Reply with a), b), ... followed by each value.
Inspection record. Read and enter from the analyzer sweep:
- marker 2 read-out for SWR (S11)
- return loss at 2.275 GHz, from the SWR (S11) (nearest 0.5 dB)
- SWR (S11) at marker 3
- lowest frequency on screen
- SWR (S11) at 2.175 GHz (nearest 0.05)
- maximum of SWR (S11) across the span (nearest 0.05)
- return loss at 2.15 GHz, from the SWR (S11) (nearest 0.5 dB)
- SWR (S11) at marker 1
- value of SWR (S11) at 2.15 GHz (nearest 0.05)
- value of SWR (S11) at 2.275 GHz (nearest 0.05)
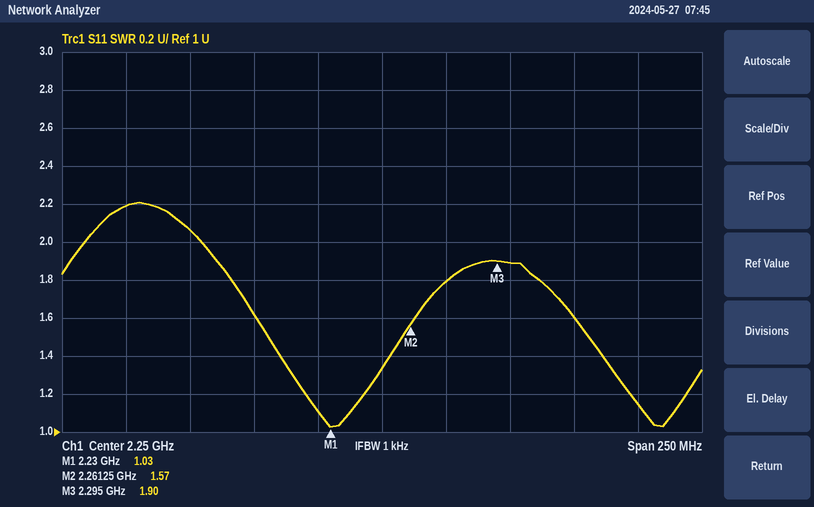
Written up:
a) 1.57
b) 11.0 dB
c) 1.90
d) 2.125 GHz
e) 2.05
f) 2.20
g) 8.5 dB
h) 1.03
i) 2.20
j) 1.80
